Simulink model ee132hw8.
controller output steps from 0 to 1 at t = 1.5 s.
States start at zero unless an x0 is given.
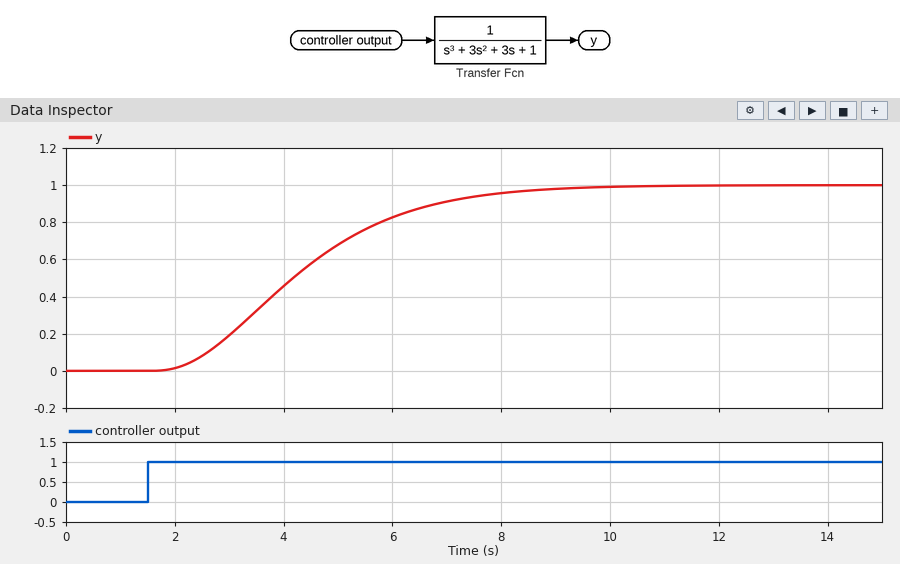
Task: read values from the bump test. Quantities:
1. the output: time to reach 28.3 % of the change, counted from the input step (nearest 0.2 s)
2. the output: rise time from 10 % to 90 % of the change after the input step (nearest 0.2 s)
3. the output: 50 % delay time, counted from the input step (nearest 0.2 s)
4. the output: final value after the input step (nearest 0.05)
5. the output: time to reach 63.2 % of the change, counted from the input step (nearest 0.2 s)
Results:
1.8 s
4.2 s
2.6 s
1.00
3.2 s
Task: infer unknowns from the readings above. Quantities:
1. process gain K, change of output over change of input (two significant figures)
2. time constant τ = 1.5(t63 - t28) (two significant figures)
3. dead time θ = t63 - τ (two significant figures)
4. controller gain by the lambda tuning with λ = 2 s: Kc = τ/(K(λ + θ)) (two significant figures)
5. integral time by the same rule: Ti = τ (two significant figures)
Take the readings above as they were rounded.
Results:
1.0
2.1 s
1.1 s
0.68
2.1 s
